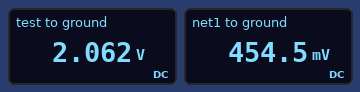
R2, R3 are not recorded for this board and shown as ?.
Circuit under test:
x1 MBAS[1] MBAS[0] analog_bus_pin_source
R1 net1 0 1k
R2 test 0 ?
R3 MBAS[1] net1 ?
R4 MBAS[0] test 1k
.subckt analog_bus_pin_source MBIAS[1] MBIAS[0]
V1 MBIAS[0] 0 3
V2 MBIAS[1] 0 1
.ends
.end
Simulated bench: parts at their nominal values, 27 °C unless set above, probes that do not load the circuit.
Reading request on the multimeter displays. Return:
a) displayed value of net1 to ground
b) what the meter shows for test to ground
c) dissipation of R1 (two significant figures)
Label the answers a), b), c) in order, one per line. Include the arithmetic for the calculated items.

a) 454.5 mV
b) 2.062 V
c) (454.5 mV)^2 / 1 kΩ = 210 µW
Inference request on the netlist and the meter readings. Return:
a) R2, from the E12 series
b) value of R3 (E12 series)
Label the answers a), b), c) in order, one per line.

a) 2.2 kΩ
b) 1.2 kΩ
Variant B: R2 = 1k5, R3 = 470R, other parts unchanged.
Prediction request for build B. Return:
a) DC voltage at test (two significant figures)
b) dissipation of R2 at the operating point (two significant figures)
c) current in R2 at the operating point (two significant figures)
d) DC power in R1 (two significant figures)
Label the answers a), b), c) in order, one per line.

a) 1.8 V
b) 2.2 mW
c) 1.2 mA
d) 460 µW
